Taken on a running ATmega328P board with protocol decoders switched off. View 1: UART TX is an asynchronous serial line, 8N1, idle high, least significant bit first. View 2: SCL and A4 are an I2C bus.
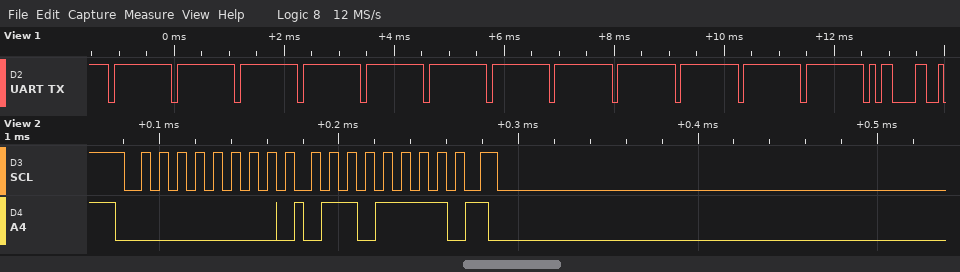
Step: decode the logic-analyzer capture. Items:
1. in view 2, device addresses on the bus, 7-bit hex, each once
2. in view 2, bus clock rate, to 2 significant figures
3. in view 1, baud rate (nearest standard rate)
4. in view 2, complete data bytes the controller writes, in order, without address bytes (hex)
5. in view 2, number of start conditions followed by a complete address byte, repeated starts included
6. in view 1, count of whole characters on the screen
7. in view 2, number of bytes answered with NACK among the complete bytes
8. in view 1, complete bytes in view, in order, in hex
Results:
0x00
100 kHz
9600 baud
6F
1
13
0
FF FF FF FF FF FF FF FF FF FF FF FF 0D
